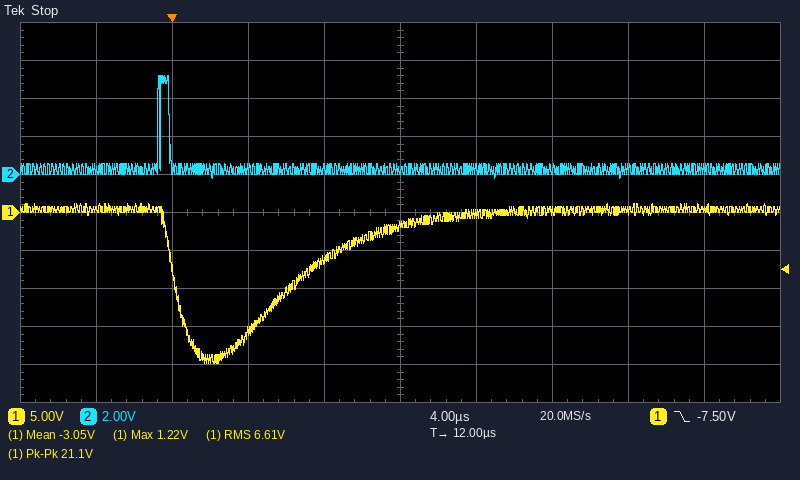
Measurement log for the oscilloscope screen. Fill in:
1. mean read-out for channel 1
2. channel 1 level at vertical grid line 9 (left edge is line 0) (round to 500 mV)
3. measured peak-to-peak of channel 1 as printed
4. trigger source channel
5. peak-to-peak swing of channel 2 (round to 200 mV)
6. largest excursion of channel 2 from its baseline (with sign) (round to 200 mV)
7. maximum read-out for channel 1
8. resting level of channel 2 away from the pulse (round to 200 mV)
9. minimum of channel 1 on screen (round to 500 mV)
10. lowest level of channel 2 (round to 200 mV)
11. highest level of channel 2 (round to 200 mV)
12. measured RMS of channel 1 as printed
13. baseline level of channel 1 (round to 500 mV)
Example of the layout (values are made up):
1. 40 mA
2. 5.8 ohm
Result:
1. -3.05 V
2. 500 mV
3. 21.1 V
4. channel 1
5. 5.4 V
6. +5.0 V
7. 1.22 V
8. 200 mV
9. -20.0 V
10. -200 mV
11. 5.2 V
12. 6.61 V
13. 500 mV
